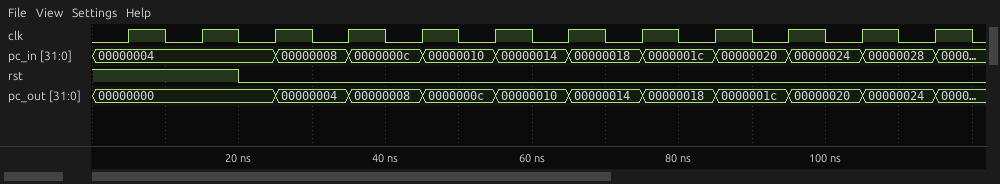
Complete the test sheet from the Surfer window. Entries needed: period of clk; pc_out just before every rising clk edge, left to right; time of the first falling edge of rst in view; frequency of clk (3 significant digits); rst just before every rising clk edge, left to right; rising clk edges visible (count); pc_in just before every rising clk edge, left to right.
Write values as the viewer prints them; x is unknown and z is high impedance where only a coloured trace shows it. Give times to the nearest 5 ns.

10 ns
00000000, 00000000, 00000000, 00000004, 00000008, 0000000c, 00000010, 00000014, 00000018, 0000001c, 00000020, 00000024
20 ns
100 MHz
1 1 0 0 0 0 0 0 0 0 0 0
12
00000004, 00000004, 00000004, 00000008, 0000000c, 00000010, 00000014, 00000018, 0000001c, 00000020, 00000024, 00000028
